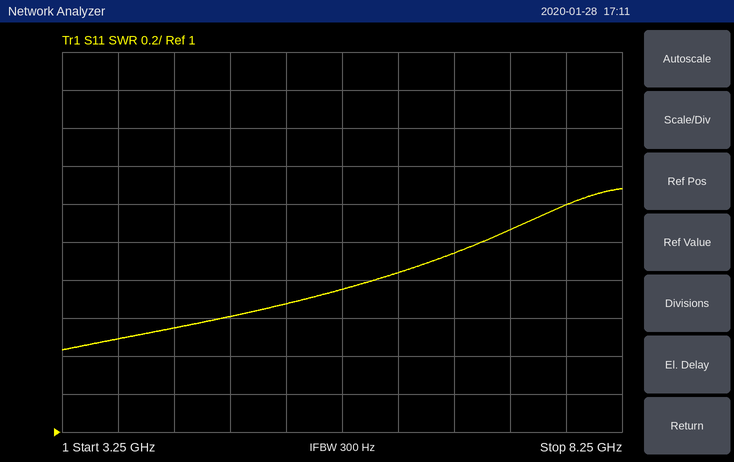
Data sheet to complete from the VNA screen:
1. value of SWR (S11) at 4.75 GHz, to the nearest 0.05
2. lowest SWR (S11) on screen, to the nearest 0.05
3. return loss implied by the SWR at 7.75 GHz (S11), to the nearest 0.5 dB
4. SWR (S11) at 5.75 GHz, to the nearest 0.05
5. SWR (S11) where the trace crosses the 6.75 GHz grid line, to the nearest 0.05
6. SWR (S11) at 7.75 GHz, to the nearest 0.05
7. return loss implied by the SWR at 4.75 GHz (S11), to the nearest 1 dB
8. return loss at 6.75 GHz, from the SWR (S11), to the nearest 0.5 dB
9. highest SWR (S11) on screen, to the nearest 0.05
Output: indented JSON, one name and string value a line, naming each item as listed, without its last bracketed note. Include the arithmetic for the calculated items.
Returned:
{
  "value of SWR (S11) at 4.75 GHz, to the nearest 0.05": "1.60",
  "lowest SWR (S11) on screen, to the nearest 0.05": "1.45",
  "return loss implied by the SWR at 7.75 GHz (S11), to the nearest 0.5 dB": "−20 log10((2.2 − 1)/(2.2 + 1)) ≈ 8.5 dB",
  "SWR (S11) at 5.75 GHz, to the nearest 0.05": "1.75",
  "SWR (S11) where the trace crosses the 6.75 GHz grid line, to the nearest 0.05": "1.95",
  "SWR (S11) at 7.75 GHz, to the nearest 0.05": "2.20",
  "return loss implied by the SWR at 4.75 GHz (S11), to the nearest 1 dB": "−20 log10((1.6 − 1)/(1.6 + 1)) ≈ 13 dB",
  "return loss at 6.75 GHz, from the SWR (S11), to the nearest 0.5 dB": "−20 log10((1.95 − 1)/(1.95 + 1)) ≈ 9.84 dB, so 10.0 dB to the nearest 0.5 dB",
  "highest SWR (S11) on screen, to the nearest 0.05": "2.30"
}
